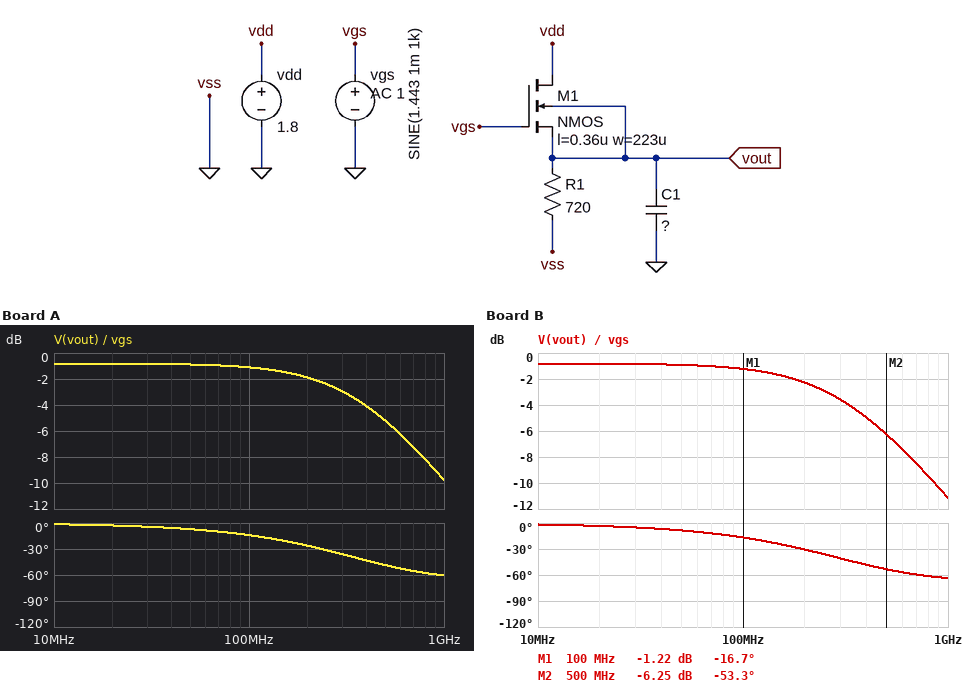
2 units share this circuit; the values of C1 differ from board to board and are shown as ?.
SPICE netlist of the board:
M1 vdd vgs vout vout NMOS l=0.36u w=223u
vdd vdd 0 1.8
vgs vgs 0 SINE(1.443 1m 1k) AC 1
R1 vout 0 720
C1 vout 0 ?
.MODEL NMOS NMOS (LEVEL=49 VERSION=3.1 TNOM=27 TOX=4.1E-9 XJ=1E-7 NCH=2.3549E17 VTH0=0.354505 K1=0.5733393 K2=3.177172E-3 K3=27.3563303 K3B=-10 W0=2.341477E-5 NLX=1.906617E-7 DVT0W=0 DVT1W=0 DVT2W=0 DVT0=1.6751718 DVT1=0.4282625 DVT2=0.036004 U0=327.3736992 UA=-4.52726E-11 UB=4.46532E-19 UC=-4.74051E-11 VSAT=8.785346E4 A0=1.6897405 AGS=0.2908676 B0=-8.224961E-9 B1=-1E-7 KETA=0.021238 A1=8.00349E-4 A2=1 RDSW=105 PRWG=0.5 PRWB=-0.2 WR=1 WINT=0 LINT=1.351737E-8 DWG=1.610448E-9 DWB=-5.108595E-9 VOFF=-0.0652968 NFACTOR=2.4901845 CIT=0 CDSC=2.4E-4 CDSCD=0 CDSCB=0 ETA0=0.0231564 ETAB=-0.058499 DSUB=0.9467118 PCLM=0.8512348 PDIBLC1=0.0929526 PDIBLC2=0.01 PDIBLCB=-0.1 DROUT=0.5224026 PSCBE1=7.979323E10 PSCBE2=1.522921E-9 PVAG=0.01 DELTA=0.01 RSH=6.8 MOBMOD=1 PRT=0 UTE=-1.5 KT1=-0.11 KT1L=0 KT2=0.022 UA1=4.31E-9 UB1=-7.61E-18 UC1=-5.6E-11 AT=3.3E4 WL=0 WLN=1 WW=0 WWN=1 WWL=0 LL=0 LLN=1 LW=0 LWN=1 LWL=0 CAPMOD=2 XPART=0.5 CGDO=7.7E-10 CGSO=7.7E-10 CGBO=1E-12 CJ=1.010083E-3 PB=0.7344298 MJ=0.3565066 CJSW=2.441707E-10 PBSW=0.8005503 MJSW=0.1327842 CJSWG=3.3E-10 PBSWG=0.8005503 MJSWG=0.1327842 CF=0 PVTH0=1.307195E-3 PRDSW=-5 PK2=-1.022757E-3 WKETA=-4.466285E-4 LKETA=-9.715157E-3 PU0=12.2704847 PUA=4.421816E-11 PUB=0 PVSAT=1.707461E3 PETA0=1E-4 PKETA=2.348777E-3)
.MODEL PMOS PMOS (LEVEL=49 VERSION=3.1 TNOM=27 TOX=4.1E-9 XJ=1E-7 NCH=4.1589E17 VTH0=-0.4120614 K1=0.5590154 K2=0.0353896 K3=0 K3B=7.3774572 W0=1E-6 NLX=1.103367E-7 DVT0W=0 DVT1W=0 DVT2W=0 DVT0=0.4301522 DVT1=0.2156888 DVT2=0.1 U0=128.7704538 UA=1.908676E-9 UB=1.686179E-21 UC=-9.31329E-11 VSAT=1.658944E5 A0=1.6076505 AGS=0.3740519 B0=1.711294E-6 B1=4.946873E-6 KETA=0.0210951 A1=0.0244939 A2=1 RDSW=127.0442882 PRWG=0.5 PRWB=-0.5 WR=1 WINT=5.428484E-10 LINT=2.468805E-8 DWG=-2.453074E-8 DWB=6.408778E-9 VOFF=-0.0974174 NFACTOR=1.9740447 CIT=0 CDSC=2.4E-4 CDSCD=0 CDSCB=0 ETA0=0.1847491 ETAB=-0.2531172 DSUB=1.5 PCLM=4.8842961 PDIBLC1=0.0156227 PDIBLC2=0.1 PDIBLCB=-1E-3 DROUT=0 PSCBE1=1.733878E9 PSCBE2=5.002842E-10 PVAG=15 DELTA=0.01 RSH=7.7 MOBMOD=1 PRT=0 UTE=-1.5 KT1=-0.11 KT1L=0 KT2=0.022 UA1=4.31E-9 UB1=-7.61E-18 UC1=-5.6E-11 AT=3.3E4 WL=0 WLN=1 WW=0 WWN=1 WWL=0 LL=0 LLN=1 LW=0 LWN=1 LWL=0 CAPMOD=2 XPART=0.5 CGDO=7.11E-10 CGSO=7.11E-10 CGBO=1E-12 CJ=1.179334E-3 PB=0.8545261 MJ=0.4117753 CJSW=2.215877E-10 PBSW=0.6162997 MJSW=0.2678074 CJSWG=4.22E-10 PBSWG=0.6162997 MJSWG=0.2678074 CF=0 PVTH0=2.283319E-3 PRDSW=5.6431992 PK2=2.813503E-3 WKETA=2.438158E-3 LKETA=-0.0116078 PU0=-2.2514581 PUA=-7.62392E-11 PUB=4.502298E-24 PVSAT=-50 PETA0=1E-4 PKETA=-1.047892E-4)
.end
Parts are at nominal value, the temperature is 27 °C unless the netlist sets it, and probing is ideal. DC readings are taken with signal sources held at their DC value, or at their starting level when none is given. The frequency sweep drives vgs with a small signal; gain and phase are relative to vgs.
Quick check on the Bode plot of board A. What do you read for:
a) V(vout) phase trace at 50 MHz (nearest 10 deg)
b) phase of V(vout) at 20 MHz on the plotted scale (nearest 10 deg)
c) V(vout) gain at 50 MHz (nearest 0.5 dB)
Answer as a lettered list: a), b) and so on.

a) -10 deg
b) 0 deg
c) -1.0 dB
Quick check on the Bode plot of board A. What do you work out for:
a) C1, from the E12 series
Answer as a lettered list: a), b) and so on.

a) 6.8 pF
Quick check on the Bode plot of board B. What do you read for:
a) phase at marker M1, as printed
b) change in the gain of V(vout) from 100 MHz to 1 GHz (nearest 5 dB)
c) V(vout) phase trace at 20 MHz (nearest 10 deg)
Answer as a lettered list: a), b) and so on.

a) -16.7 deg
b) -10 dB
c) 0 deg
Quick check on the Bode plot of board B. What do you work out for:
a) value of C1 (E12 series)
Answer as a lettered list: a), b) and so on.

a) 8.2 pF
